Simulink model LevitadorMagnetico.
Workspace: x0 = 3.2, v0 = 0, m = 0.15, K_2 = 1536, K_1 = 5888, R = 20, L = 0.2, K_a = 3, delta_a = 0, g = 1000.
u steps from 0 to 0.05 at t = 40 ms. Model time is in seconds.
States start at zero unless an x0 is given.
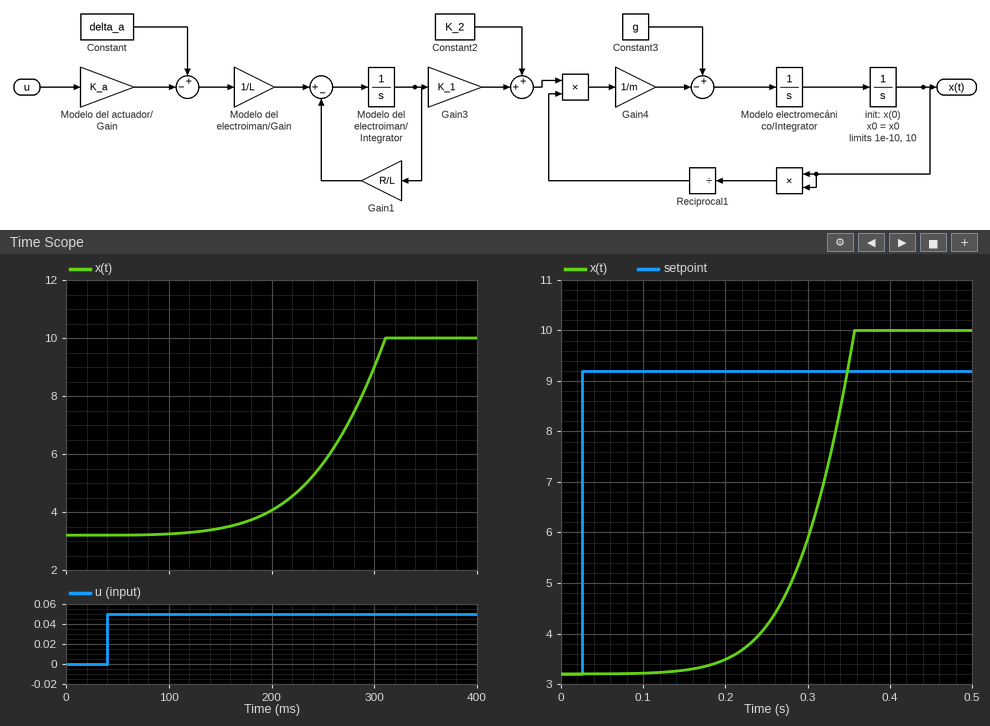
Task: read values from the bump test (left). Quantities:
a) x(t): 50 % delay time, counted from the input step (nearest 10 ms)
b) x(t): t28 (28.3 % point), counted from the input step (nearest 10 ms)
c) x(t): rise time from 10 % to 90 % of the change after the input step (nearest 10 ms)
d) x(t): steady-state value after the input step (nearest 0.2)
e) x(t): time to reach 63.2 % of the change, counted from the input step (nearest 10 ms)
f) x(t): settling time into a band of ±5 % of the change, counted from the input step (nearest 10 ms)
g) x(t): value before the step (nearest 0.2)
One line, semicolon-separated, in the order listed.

230 ms; 200 ms; 110 ms; 10.0; 240 ms; 270 ms; 3.2
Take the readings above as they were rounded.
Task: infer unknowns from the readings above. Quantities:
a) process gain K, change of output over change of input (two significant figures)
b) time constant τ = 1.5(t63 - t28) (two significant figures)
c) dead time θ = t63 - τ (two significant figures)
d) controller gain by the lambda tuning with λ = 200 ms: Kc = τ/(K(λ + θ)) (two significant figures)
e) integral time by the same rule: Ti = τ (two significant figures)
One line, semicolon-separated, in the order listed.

140; 60 ms; 180 ms; 0.0011; 60 ms
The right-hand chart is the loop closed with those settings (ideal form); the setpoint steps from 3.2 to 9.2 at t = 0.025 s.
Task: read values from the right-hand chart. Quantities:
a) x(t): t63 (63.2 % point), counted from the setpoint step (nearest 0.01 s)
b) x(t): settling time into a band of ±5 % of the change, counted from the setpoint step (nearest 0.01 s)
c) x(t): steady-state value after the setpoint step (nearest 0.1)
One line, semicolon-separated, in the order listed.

0.30 s; 0.33 s; 10.0
